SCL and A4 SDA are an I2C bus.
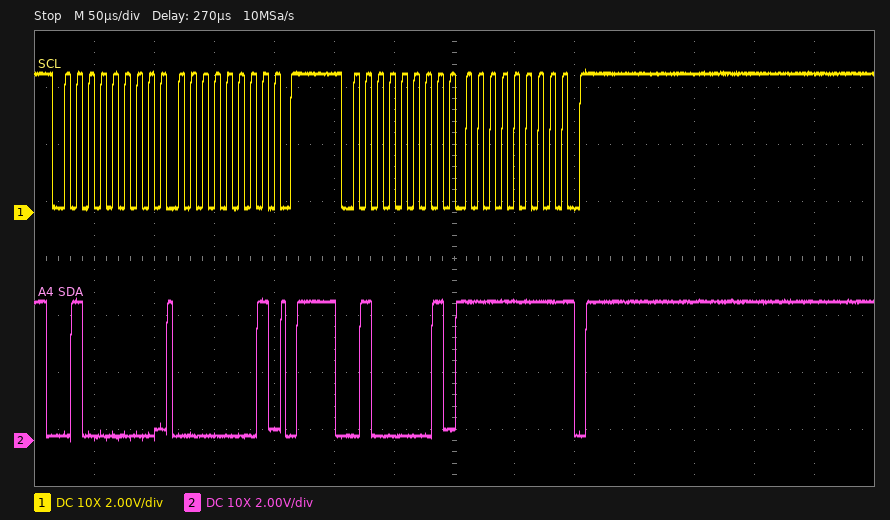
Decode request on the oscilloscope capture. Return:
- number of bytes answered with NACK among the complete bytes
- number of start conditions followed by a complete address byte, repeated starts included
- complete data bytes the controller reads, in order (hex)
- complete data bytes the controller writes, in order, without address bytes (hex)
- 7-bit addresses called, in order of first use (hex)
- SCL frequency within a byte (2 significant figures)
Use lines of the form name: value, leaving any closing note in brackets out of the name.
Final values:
number of bytes answered with NACK among the complete bytes: 1
number of start conditions followed by a complete address byte, repeated starts included: 2
complete data bytes the controller reads, in order: FF
complete data bytes the controller writes, in order, without address bytes: 01
7-bit addresses called, in order of first use: 0x20
SCL frequency within a byte: 100 kHz
